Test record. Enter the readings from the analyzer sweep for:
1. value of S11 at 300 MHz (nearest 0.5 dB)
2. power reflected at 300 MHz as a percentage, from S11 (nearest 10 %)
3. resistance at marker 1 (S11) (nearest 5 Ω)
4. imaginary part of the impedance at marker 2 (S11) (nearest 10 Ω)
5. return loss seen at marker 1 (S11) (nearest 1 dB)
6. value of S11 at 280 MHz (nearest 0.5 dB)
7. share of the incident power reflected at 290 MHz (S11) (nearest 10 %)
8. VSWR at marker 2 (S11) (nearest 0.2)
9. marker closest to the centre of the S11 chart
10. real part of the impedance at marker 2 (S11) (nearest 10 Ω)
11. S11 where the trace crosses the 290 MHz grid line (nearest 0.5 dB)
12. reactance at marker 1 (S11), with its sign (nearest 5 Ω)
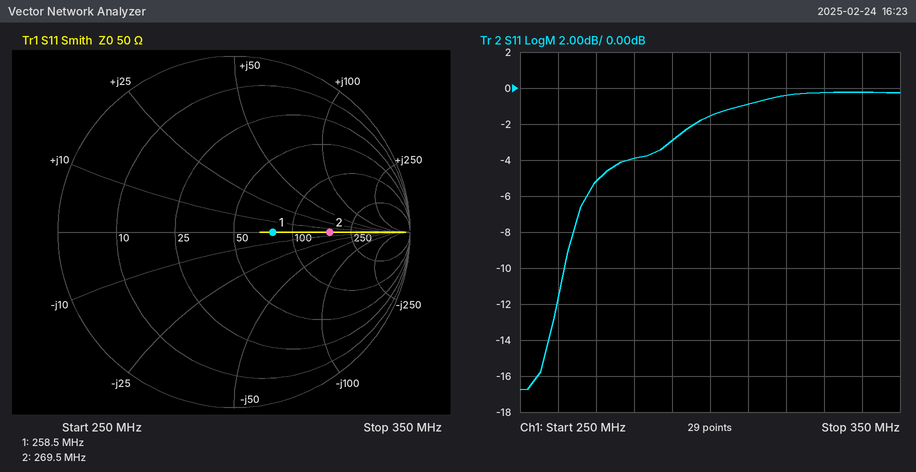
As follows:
-1.5 dB
70 %
80 Ω
0 Ω
13 dB
-4.0 dB
50 %
3.4
marker 1
170 Ω
-3.0 dB
0 Ω
